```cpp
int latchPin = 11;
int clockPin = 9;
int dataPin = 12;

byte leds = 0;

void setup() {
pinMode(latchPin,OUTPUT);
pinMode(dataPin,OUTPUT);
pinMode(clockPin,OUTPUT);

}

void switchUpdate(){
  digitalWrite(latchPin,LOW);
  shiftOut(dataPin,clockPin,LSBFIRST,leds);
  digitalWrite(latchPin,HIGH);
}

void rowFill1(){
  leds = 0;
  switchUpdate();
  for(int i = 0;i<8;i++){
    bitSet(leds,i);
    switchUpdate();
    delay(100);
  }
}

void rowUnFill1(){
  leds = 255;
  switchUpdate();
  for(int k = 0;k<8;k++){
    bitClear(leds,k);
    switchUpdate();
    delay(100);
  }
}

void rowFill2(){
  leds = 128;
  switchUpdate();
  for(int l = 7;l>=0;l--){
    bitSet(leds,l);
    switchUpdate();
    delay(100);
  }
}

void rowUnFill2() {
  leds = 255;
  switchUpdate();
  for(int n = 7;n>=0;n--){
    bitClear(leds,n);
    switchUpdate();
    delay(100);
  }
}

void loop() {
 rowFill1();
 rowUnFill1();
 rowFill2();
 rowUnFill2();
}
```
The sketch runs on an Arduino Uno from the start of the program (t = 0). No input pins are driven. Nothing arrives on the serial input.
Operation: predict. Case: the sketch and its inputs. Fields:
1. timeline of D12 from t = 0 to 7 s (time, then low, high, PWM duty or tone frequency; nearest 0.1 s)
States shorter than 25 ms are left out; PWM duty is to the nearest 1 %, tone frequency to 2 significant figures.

0 s low; 0.7 s high; 1.5 s low; 1.6 s high; 2.4 s low; 3.9 s high; 4.7 s low; 4.8 s high; 5.6 s low
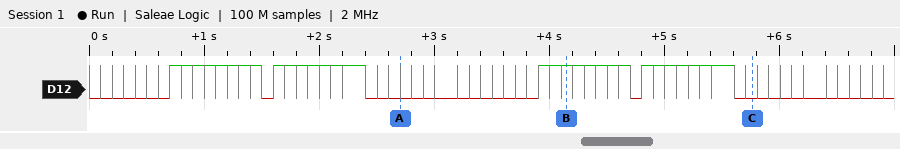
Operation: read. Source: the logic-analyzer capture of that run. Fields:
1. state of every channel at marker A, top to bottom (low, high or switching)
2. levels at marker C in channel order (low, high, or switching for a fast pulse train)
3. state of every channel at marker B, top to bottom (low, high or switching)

D12 low
D12 low
D12 high
